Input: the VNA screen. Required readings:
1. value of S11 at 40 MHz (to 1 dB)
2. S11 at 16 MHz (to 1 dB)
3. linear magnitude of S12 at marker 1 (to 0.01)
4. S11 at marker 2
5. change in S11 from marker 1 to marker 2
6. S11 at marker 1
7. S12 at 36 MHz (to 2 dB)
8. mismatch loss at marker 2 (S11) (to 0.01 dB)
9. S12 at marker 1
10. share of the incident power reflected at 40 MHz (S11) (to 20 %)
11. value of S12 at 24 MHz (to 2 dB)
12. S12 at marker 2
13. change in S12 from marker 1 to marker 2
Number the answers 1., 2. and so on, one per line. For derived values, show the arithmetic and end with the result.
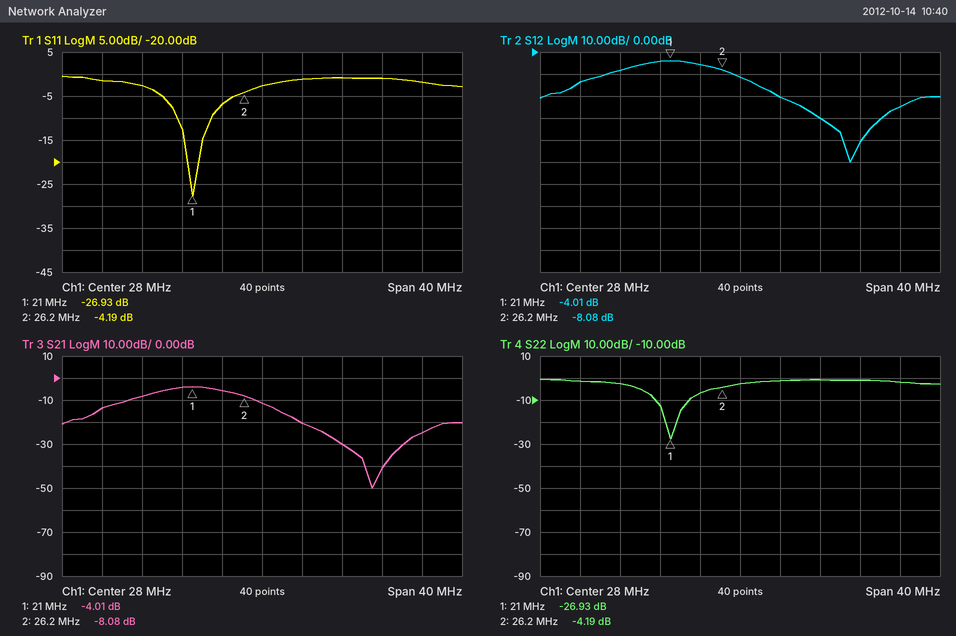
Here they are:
1. -1 dB
2. -3 dB
3. 10^(-4.01/20) ≈ 0.63
4. -4.19 dB
5. -4.19 − (-26.93) = 22.74 dB
6. -26.93 dB
7. -30 dB
8. −10 log10(1 − 10^(-4.19/10)) ≈ 2.08 dB
9. -4.01 dB
10. 10^(-1/10) ≈ 79.4 %, so 80 % to the nearest 20 %
11. -6 dB
12. -8.08 dB
13. -8.08 − (-4.01) = -4.07 dB
